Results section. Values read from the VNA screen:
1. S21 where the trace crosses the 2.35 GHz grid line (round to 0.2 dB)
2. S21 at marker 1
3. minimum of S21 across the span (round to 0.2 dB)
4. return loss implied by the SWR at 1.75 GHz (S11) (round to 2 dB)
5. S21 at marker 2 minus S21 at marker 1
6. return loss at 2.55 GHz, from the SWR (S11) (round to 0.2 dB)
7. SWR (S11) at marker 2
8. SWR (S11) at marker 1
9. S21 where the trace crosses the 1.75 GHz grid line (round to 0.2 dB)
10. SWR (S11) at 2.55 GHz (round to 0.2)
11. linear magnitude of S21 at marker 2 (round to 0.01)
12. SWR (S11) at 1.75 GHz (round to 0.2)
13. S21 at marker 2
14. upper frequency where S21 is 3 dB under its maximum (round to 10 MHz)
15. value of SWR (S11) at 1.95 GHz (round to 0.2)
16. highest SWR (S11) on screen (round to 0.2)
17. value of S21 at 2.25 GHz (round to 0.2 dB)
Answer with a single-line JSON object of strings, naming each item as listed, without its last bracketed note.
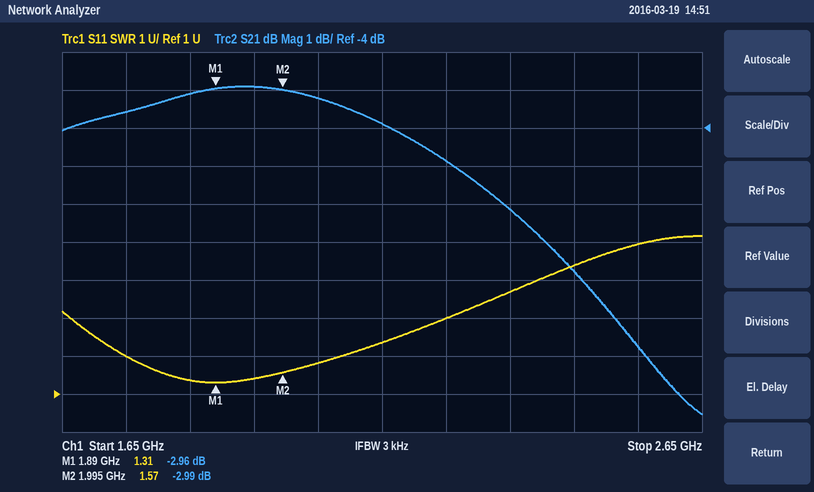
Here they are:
{"S21 where the trace crosses the 2.35 GHz grid line": "-6.2 dB", "S21 at marker 1": "-2.96 dB", "minimum of S21 across the span": "-11.6 dB", "return loss implied by the SWR at 1.75 GHz (S11)": "10 dB", "S21 at marker 2 minus S21 at marker 1": "-0.03 dB", "return loss at 2.55 GHz, from the SWR (S11)": "3.6 dB", "SWR (S11) at marker 2": "1.57", "SWR (S11) at marker 1": "1.31", "S21 where the trace crosses the 1.75 GHz grid line": "-3.6 dB", "SWR (S11) at 2.55 GHz": "5.0", "linear magnitude of S21 at marker 2": "0.71", "SWR (S11) at 1.75 GHz": "2.0", "S21 at marker 2": "-2.99 dB", "upper frequency where S21 is 3 dB under its maximum": "2.33 GHz", "value of SWR (S11) at 1.95 GHz": "1.4", "highest SWR (S11) on screen": "5.2", "value of S21 at 2.25 GHz": "-4.8 dB"}
